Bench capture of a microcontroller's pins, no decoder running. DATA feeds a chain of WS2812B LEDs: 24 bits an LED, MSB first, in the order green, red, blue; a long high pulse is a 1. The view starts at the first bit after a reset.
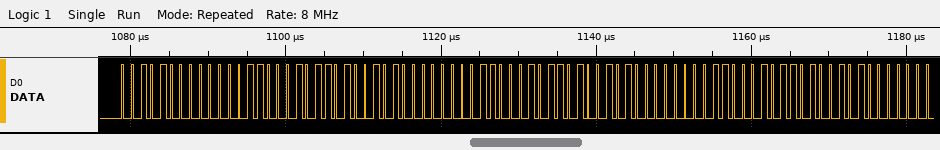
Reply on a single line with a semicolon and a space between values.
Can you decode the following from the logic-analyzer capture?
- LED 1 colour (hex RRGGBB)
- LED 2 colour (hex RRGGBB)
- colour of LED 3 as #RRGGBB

#06282D; #06282D; #06282D
